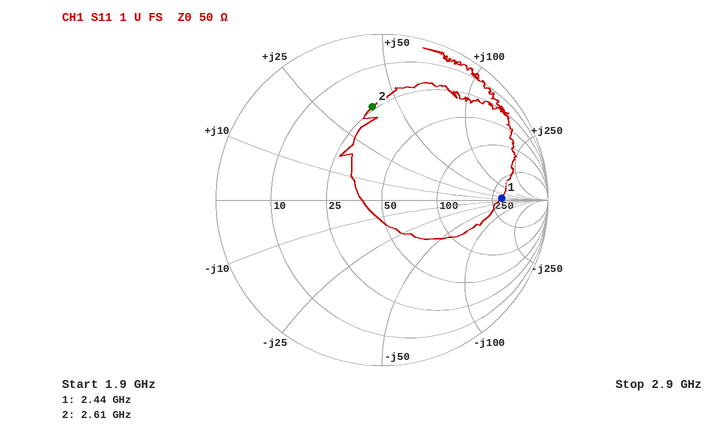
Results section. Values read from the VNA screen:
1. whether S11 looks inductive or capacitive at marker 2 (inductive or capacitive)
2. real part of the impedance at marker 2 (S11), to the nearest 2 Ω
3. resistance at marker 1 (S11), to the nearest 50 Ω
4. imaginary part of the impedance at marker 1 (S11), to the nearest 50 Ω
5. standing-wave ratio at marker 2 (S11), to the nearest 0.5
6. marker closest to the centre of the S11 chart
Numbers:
inductive
24 Ω
300 Ω
0 Ω
3.5
marker 2
